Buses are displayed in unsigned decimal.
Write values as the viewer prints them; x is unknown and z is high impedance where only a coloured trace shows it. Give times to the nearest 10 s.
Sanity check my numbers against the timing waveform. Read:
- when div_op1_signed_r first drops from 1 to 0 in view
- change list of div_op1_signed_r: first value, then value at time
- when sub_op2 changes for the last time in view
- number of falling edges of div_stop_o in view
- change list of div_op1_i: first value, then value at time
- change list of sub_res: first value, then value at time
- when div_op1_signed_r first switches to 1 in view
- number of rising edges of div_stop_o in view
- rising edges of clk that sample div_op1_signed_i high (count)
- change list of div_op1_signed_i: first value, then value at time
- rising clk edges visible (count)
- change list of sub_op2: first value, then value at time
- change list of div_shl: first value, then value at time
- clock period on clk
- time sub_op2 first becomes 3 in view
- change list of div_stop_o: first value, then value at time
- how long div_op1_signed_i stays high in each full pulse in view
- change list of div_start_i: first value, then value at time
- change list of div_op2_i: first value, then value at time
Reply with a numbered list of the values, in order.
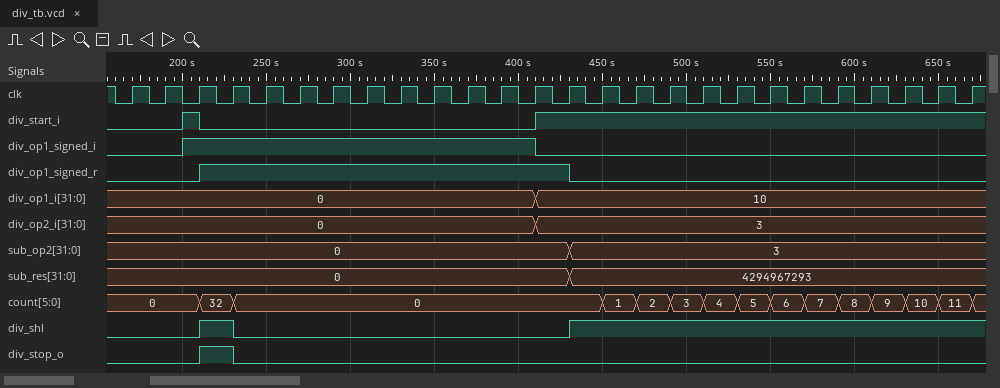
1. 430 s
2. 0, 1 at 210 s, 0 at 430 s
3. 430 s
4. 1
5. 0, 10 at 410 s
6. 0, 4294967293 at 430 s
7. 210 s
8. 1
9. 11
10. 0, 1 at 200 s, 0 at 410 s
11. 26
12. 0, 3 at 430 s
13. 0, 1 at 210 s, 0 at 230 s, 1 at 430 s
14. 20 s
15. 430 s
16. 0, 1 at 210 s, 0 at 230 s
17. 210 s
18. 0, 1 at 200 s, 0 at 210 s, 1 at 410 s
19. 0, 3 at 410 s
